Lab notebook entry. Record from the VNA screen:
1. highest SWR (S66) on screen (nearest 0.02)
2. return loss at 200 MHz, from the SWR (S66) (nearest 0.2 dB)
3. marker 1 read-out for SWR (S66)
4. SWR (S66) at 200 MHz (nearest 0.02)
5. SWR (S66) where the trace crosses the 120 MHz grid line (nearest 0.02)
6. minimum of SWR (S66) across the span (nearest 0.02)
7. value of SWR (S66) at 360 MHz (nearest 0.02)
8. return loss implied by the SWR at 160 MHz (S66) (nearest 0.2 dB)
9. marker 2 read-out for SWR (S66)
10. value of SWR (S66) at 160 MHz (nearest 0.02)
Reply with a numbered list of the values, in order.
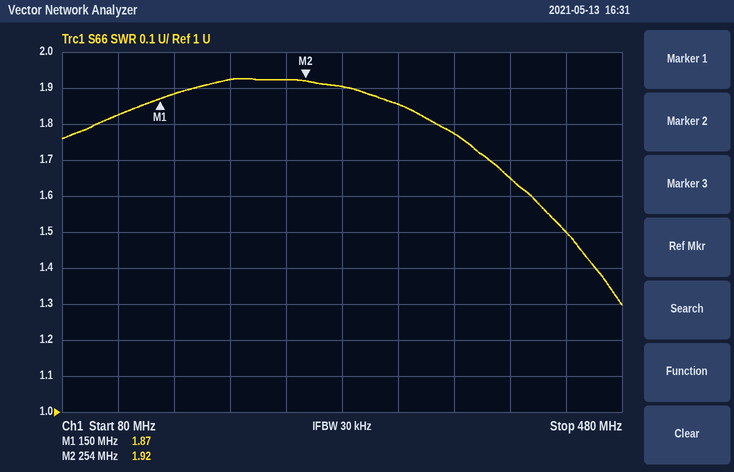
1. 1.92
2. 10.0 dB
3. 1.87
4. 1.92
5. 1.82
6. 1.30
7. 1.78
8. 10.2 dB
9. 1.92
10. 1.88
